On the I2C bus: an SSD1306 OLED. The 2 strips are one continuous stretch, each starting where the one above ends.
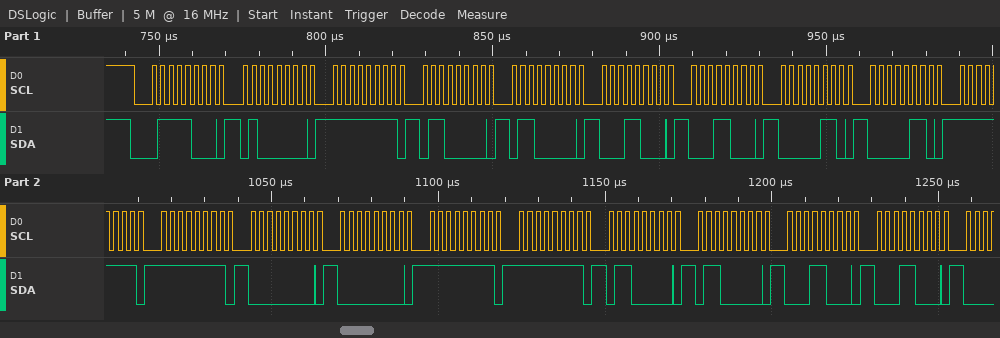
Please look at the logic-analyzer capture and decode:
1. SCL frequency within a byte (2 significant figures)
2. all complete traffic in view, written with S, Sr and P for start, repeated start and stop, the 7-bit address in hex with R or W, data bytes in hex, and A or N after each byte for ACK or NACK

400 kHz
S 3CW A 40 A FF A 60 A 60 A 18 A 18 A 06 A 06 A FF A FF A 00 A 00 A FF A FF A 60 A 60 A 18 A 18 A
